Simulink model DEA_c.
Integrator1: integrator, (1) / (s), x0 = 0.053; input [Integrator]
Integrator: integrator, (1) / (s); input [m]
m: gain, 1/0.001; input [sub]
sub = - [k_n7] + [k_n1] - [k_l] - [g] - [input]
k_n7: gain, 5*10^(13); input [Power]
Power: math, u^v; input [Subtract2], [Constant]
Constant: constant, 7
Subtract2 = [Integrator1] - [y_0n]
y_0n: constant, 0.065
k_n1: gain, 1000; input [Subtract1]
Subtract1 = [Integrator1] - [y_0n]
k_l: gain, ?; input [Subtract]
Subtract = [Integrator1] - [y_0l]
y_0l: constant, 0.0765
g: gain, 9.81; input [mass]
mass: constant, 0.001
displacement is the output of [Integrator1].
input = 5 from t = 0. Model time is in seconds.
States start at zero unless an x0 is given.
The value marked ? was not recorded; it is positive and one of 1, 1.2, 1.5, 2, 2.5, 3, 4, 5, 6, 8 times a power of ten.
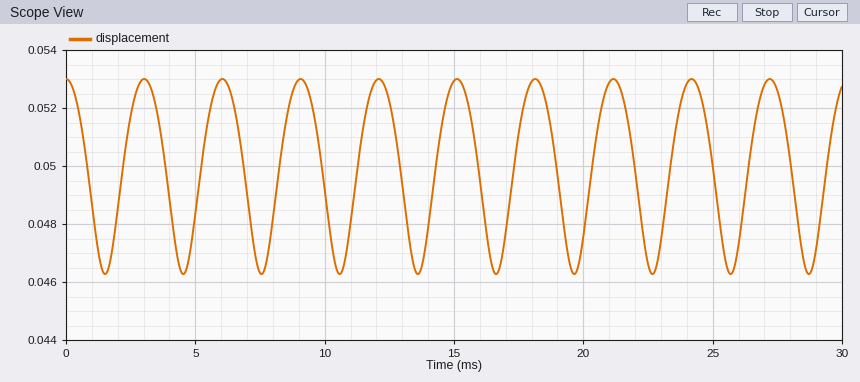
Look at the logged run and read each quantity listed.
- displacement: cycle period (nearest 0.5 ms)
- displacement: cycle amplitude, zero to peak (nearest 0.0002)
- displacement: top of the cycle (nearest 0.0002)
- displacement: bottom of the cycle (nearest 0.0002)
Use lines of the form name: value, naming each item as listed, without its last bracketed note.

displacement: cycle period: 3.0 ms
displacement: cycle amplitude, zero to peak: 0.0034
displacement: top of the cycle: 0.0530
displacement: bottom of the cycle: 0.0462
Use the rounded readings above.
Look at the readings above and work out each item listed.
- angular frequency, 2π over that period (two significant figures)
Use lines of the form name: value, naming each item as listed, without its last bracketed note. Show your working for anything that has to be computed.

angular frequency, 2π over that period: 2π / 3 = 2.1 rad/ms
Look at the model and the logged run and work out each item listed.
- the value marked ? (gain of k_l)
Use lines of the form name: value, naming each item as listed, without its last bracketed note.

the value marked ?: 250
